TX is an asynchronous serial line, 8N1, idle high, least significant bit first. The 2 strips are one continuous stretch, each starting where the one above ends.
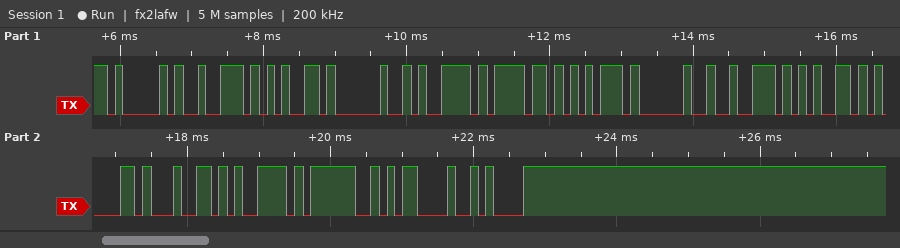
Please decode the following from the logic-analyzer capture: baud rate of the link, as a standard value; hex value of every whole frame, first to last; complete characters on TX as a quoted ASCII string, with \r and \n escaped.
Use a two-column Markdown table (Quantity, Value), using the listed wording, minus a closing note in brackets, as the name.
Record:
| Quantity | Value |
|---|---|
| baud rate of the link, as a standard value | 9600 baud |
| hex value of every whole frame, first to last | 41 72 65 20 79 6F 75 20 72 65 61 64 79 3F 0D 0A |
| complete characters on TX as a quoted ASCII string, with \r and \n escaped | "Are you ready?\r\n" |
